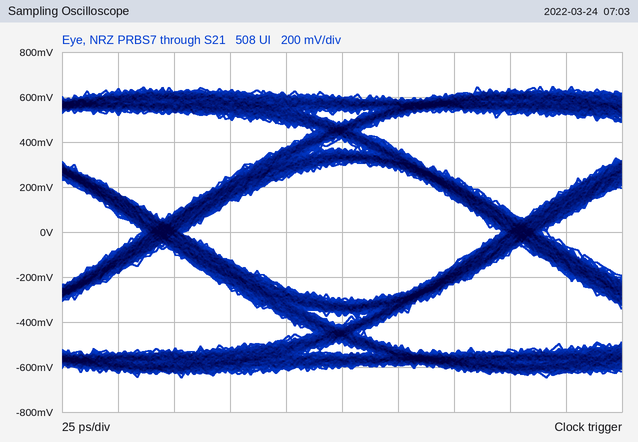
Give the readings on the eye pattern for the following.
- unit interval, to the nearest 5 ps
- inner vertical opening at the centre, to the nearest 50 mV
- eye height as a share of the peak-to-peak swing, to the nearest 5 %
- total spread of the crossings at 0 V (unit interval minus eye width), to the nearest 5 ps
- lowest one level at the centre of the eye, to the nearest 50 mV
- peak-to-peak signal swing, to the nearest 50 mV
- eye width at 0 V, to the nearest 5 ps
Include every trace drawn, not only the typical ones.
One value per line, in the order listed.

160 ps
600 mV
45 %
20 ps
300 mV
1.30 V
140 ps
